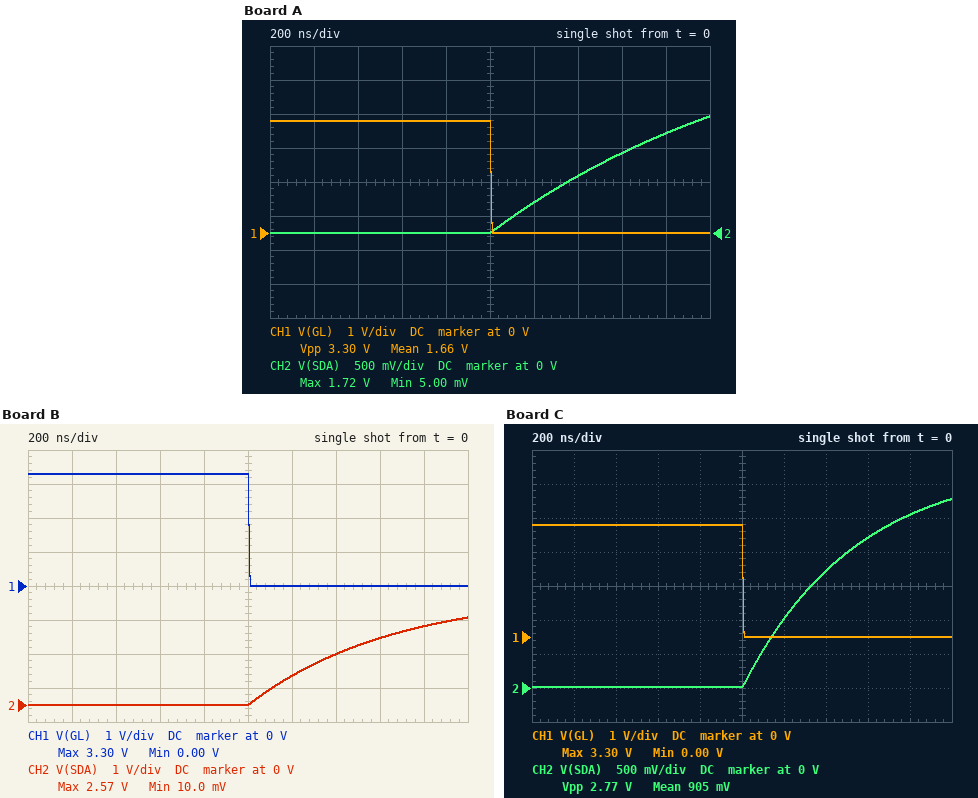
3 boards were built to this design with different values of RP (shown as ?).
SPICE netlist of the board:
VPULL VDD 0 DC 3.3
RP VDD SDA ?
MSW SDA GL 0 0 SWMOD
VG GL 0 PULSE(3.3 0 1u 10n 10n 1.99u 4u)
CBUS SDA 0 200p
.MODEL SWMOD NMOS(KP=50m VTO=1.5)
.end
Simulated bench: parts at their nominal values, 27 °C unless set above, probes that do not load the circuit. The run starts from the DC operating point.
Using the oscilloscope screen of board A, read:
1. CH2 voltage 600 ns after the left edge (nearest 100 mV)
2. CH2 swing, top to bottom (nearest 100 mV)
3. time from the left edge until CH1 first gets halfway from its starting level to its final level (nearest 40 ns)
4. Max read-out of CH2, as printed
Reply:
0 V
1.7 V
1.00 µs
1.72 V
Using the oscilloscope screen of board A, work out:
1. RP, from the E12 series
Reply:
6.8 kΩ
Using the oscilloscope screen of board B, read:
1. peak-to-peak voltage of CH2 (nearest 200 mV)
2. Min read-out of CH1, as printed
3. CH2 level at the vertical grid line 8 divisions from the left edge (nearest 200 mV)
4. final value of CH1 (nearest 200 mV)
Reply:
2.6 V
0.00 V
2.0 V
0 V
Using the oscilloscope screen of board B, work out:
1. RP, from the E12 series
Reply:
3.3 kΩ
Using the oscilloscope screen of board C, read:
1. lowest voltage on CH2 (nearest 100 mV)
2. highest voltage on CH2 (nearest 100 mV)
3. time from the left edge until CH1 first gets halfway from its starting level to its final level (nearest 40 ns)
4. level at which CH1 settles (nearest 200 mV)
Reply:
0 V
2.8 V
1.00 µs
0 V
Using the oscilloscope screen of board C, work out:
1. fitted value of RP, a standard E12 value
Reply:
2.7 kΩ
